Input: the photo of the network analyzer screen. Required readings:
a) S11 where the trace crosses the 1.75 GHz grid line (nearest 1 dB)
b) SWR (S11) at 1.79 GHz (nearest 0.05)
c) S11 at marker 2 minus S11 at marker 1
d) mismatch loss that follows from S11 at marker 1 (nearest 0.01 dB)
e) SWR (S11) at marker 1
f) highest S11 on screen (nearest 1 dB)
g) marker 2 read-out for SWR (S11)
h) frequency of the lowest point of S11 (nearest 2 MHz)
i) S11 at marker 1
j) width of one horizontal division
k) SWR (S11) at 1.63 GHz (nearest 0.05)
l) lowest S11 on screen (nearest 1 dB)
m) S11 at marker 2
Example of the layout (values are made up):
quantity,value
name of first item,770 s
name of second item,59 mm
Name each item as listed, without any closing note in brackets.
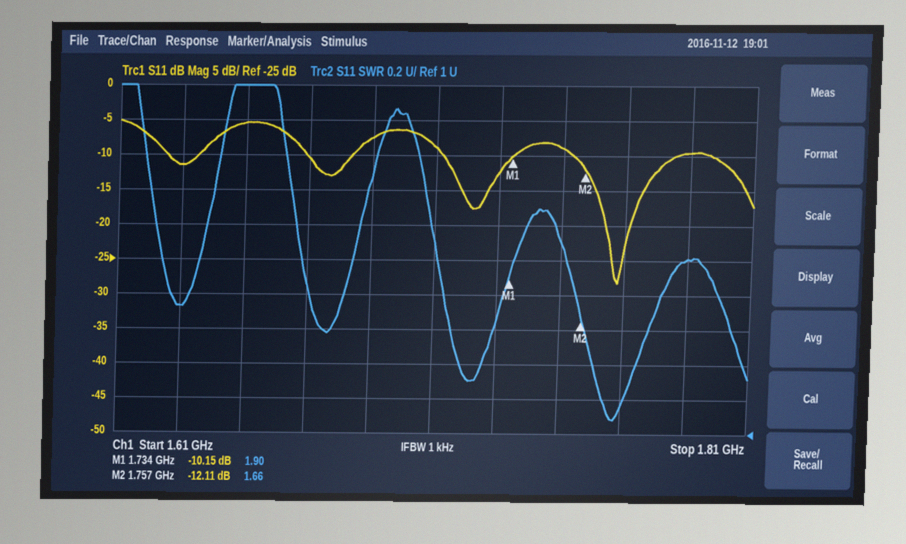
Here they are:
quantity,value
S11 where the trace crosses the 1.75 GHz grid line,-9 dB
SWR (S11) at 1.79 GHz,2.00
S11 at marker 2 minus S11 at marker 1,-1.96 dB
mismatch loss that follows from S11 at marker 1,0.44 dB
SWR (S11) at marker 1,1.90
highest S11 on screen,-5 dB
marker 2 read-out for SWR,1.66
frequency of the lowest point of S11,1.768 GHz
S11 at marker 1,-10.15 dB
width of one horizontal division,20 MHz
SWR (S11) at 1.63 GHz,1.75
lowest S11 on screen,-28 dB
S11 at marker 2,-12.11 dB
